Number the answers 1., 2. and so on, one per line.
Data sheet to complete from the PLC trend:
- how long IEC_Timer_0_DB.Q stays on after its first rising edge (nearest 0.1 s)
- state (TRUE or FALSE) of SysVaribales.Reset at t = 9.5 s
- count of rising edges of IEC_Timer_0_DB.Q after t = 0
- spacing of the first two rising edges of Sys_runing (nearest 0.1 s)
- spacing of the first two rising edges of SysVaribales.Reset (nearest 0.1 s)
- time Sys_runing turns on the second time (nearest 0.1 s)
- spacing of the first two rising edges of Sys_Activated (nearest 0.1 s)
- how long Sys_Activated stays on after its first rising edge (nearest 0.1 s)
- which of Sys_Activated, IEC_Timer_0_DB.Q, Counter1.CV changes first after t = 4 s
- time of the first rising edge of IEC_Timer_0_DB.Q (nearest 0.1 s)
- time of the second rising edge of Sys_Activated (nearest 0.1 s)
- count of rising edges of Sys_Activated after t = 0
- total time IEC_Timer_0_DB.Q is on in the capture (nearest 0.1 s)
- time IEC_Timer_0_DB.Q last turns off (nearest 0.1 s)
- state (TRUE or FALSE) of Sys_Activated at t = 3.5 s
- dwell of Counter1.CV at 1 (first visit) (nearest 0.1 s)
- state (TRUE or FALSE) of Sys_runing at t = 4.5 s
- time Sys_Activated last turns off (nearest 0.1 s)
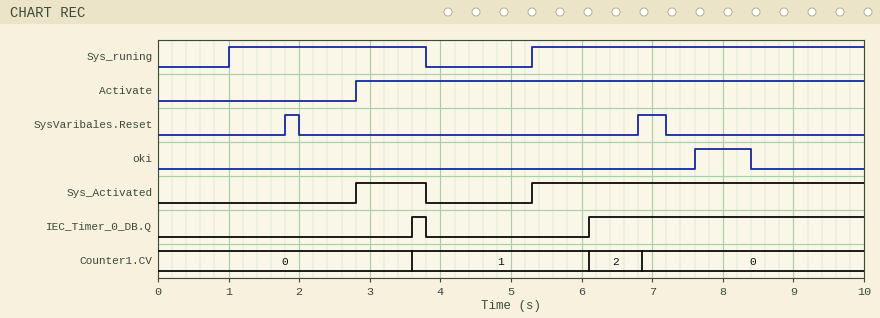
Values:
1. 0.2 s
2. FALSE
3. 2
4. 4.3 s
5. 5.0 s
6. 5.3 s
7. 2.5 s
8. 1.0 s
9. Sys_Activated
10. 3.6 s
11. 5.3 s
12. 2
13. 4.1 s
14. 3.8 s
15. TRUE
16. 2.5 s
17. FALSE
18. 3.8 s
